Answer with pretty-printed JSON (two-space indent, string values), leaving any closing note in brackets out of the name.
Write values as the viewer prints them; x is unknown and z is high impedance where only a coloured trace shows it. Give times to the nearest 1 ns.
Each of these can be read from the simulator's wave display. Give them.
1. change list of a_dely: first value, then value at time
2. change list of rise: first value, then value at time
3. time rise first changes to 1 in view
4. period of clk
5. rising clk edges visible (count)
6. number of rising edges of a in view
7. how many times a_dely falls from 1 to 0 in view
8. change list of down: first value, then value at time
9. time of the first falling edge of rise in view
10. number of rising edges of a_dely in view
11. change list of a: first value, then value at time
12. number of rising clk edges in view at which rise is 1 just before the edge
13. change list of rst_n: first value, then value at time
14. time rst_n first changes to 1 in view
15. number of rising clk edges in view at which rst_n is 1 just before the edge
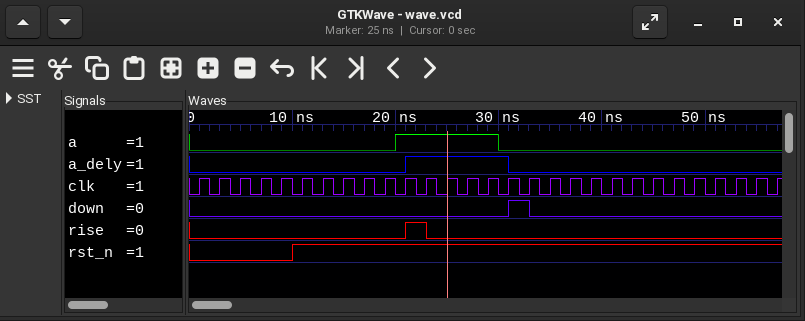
{
  "change list of a_dely: first value, then value at time": "0, 1 at 21 ns, 0 at 31 ns",
  "change list of rise: first value, then value at time": "0, 1 at 21 ns, 0 at 23 ns",
  "time rise first changes to 1 in view": "21 ns",
  "period of clk": "2 ns",
  "rising clk edges visible": "29",
  "number of rising edges of a in view": "1",
  "how many times a_dely falls from 1 to 0 in view": "1",
  "change list of down: first value, then value at time": "0, 1 at 31 ns, 0 at 33 ns",
  "time of the first falling edge of rise in view": "23 ns",
  "number of rising edges of a_dely in view": "1",
  "change list of a: first value, then value at time": "0, 1 at 20 ns, 0 at 30 ns",
  "number of rising clk edges in view at which rise is 1 just before the edge": "1",
  "change list of rst_n: first value, then value at time": "0, 1 at 10 ns",
  "time rst_n first changes to 1 in view": "10 ns",
  "number of rising clk edges in view at which rst_n is 1 just before the edge": "24"
}
